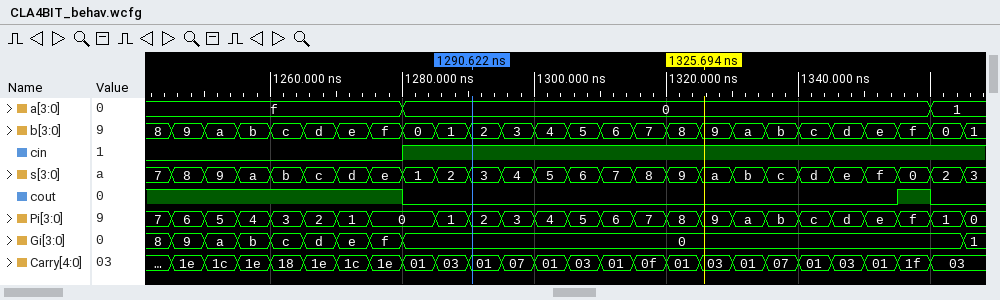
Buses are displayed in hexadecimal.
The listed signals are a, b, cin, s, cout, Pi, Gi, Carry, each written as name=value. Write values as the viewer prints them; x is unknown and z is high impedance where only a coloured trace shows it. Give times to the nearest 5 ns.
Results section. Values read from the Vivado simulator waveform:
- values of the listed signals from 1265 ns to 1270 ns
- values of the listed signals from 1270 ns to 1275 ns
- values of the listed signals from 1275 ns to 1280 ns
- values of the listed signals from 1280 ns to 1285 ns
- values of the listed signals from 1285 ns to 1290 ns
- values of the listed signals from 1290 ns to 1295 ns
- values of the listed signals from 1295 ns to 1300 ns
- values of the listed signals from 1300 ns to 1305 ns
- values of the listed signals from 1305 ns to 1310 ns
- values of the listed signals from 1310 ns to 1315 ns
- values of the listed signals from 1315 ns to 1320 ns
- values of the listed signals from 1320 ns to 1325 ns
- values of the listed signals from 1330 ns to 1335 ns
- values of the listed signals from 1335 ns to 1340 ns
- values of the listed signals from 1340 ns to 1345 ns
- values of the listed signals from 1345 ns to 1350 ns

a=f, b=d, cin=0, s=c, cout=1, Pi=2, Gi=d, Carry=1e
a=f, b=e, cin=0, s=d, cout=1, Pi=1, Gi=e, Carry=1c
a=f, b=f, cin=0, s=e, cout=1, Pi=0, Gi=f, Carry=1e
a=0, b=0, cin=1, s=1, cout=0, Pi=0, Gi=0, Carry=01
a=0, b=1, cin=1, s=2, cout=0, Pi=1, Gi=0, Carry=03
a=0, b=2, cin=1, s=3, cout=0, Pi=2, Gi=0, Carry=01
a=0, b=3, cin=1, s=4, cout=0, Pi=3, Gi=0, Carry=07
a=0, b=4, cin=1, s=5, cout=0, Pi=4, Gi=0, Carry=01
a=0, b=5, cin=1, s=6, cout=0, Pi=5, Gi=0, Carry=03
a=0, b=6, cin=1, s=7, cout=0, Pi=6, Gi=0, Carry=01
a=0, b=7, cin=1, s=8, cout=0, Pi=7, Gi=0, Carry=0f
a=0, b=8, cin=1, s=9, cout=0, Pi=8, Gi=0, Carry=01
a=0, b=a, cin=1, s=b, cout=0, Pi=a, Gi=0, Carry=01
a=0, b=b, cin=1, s=c, cout=0, Pi=b, Gi=0, Carry=07
a=0, b=c, cin=1, s=d, cout=0, Pi=c, Gi=0, Carry=01
a=0, b=d, cin=1, s=e, cout=0, Pi=d, Gi=0, Carry=03
